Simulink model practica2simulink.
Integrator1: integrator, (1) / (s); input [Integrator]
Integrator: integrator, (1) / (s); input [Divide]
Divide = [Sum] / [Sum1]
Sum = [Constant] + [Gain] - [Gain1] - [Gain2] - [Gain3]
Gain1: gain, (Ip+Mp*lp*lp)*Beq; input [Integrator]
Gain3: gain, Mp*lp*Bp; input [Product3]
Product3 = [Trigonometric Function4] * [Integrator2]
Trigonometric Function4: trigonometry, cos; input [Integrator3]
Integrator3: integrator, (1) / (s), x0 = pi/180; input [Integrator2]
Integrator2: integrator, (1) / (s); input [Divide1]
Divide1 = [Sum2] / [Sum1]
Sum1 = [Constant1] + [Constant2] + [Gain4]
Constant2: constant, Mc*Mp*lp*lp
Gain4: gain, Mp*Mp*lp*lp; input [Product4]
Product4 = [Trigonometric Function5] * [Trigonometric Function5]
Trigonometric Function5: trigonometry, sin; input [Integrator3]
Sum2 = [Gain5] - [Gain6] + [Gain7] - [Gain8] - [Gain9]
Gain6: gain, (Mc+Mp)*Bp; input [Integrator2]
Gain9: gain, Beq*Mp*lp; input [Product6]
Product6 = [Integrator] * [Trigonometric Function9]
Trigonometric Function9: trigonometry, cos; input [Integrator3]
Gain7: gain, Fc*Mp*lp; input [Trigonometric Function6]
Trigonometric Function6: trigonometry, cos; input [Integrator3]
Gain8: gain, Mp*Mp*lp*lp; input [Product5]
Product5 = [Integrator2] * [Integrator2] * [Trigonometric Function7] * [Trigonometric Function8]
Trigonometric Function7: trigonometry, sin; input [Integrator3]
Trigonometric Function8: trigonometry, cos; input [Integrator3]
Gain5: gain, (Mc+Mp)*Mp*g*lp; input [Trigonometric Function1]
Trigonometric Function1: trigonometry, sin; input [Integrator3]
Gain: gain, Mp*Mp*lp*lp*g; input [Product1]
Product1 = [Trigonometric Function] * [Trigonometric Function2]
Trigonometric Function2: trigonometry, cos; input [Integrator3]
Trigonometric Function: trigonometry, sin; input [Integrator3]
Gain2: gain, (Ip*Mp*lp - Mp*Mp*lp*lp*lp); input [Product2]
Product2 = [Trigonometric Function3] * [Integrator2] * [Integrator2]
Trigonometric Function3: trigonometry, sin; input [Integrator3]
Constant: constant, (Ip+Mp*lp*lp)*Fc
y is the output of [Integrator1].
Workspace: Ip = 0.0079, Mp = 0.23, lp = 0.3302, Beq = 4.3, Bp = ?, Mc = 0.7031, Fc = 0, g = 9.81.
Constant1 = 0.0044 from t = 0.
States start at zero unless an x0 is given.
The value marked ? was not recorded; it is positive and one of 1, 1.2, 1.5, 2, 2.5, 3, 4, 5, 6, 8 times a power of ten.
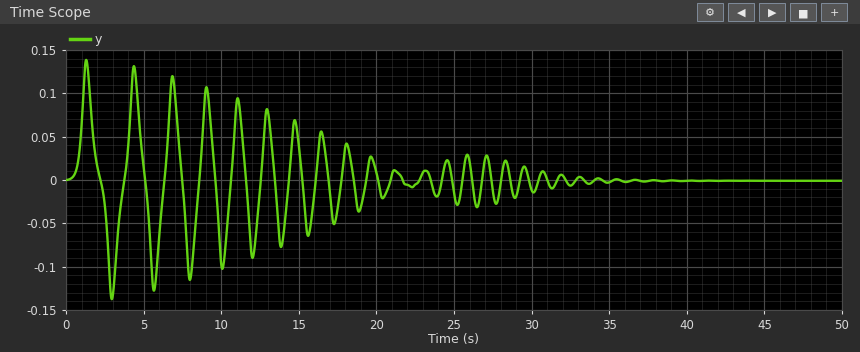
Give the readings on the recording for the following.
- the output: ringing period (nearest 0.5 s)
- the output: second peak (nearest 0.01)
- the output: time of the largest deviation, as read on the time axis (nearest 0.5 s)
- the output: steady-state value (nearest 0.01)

3.0 s
0.13
1.5 s
0.00
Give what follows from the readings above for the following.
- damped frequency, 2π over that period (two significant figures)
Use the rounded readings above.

2.1 rad/s
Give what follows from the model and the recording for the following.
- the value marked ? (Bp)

0.005
